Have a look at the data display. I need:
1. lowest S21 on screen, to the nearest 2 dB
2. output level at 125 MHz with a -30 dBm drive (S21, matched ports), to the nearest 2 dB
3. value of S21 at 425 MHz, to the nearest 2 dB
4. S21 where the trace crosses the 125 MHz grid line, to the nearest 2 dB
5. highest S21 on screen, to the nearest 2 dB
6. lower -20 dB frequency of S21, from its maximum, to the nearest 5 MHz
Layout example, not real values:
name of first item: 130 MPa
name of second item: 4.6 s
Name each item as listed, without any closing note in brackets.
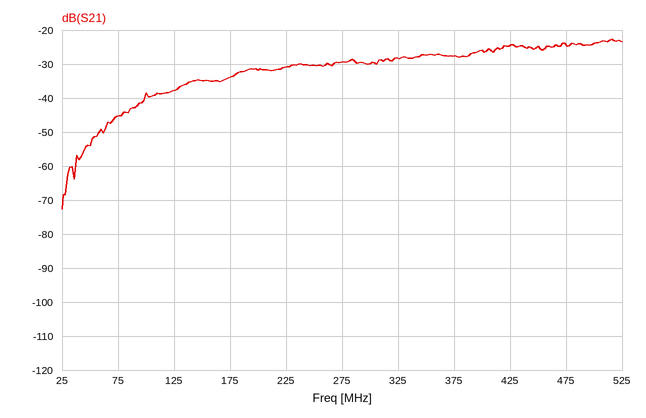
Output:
lowest S21 on screen, to the nearest 2 dB: -72 dB
output level at 125 MHz with a -30 dBm drive (S21, matched ports), to the nearest 2 dB: -68 dBm
value of S21 at 425 MHz, to the nearest 2 dB: -24 dB
S21 where the trace crosses the 125 MHz grid line, to the nearest 2 dB: -38 dB
highest S21 on screen, to the nearest 2 dB: -22 dB
lower -20 dB frequency of S21, from its maximum, to the nearest 5 MHz: 90 MHz
